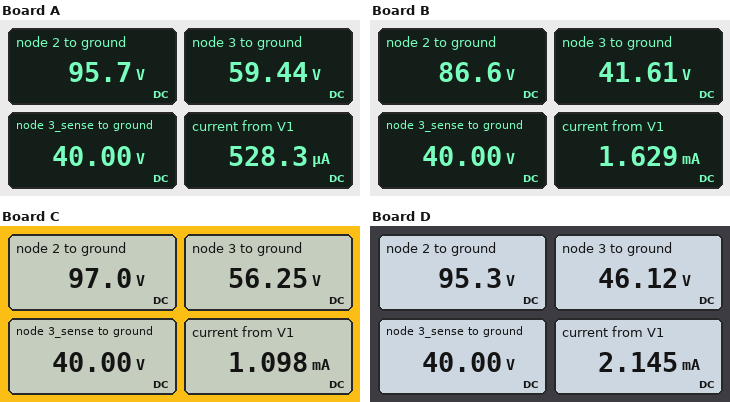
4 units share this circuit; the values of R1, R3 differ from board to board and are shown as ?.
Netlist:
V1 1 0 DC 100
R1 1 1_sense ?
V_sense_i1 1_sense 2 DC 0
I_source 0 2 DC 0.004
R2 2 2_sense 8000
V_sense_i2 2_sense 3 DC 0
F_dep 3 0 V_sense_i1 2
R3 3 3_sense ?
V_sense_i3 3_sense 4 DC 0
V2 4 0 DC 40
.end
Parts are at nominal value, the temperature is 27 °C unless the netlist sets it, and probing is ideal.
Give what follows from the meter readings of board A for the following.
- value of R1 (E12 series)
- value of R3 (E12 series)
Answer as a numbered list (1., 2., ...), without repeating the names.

1. 8.2 kΩ
2. 5.6 kΩ
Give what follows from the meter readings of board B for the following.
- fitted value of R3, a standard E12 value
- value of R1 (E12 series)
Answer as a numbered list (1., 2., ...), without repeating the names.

1. 680 Ω
2. 8.2 kΩ
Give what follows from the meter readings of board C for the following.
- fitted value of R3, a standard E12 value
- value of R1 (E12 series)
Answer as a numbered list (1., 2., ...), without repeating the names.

1. 5.6 kΩ
2. 2.7 kΩ
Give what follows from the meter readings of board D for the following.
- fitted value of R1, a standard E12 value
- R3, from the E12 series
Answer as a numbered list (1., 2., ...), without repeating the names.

1. 2.2 kΩ
2. 3.3 kΩ
